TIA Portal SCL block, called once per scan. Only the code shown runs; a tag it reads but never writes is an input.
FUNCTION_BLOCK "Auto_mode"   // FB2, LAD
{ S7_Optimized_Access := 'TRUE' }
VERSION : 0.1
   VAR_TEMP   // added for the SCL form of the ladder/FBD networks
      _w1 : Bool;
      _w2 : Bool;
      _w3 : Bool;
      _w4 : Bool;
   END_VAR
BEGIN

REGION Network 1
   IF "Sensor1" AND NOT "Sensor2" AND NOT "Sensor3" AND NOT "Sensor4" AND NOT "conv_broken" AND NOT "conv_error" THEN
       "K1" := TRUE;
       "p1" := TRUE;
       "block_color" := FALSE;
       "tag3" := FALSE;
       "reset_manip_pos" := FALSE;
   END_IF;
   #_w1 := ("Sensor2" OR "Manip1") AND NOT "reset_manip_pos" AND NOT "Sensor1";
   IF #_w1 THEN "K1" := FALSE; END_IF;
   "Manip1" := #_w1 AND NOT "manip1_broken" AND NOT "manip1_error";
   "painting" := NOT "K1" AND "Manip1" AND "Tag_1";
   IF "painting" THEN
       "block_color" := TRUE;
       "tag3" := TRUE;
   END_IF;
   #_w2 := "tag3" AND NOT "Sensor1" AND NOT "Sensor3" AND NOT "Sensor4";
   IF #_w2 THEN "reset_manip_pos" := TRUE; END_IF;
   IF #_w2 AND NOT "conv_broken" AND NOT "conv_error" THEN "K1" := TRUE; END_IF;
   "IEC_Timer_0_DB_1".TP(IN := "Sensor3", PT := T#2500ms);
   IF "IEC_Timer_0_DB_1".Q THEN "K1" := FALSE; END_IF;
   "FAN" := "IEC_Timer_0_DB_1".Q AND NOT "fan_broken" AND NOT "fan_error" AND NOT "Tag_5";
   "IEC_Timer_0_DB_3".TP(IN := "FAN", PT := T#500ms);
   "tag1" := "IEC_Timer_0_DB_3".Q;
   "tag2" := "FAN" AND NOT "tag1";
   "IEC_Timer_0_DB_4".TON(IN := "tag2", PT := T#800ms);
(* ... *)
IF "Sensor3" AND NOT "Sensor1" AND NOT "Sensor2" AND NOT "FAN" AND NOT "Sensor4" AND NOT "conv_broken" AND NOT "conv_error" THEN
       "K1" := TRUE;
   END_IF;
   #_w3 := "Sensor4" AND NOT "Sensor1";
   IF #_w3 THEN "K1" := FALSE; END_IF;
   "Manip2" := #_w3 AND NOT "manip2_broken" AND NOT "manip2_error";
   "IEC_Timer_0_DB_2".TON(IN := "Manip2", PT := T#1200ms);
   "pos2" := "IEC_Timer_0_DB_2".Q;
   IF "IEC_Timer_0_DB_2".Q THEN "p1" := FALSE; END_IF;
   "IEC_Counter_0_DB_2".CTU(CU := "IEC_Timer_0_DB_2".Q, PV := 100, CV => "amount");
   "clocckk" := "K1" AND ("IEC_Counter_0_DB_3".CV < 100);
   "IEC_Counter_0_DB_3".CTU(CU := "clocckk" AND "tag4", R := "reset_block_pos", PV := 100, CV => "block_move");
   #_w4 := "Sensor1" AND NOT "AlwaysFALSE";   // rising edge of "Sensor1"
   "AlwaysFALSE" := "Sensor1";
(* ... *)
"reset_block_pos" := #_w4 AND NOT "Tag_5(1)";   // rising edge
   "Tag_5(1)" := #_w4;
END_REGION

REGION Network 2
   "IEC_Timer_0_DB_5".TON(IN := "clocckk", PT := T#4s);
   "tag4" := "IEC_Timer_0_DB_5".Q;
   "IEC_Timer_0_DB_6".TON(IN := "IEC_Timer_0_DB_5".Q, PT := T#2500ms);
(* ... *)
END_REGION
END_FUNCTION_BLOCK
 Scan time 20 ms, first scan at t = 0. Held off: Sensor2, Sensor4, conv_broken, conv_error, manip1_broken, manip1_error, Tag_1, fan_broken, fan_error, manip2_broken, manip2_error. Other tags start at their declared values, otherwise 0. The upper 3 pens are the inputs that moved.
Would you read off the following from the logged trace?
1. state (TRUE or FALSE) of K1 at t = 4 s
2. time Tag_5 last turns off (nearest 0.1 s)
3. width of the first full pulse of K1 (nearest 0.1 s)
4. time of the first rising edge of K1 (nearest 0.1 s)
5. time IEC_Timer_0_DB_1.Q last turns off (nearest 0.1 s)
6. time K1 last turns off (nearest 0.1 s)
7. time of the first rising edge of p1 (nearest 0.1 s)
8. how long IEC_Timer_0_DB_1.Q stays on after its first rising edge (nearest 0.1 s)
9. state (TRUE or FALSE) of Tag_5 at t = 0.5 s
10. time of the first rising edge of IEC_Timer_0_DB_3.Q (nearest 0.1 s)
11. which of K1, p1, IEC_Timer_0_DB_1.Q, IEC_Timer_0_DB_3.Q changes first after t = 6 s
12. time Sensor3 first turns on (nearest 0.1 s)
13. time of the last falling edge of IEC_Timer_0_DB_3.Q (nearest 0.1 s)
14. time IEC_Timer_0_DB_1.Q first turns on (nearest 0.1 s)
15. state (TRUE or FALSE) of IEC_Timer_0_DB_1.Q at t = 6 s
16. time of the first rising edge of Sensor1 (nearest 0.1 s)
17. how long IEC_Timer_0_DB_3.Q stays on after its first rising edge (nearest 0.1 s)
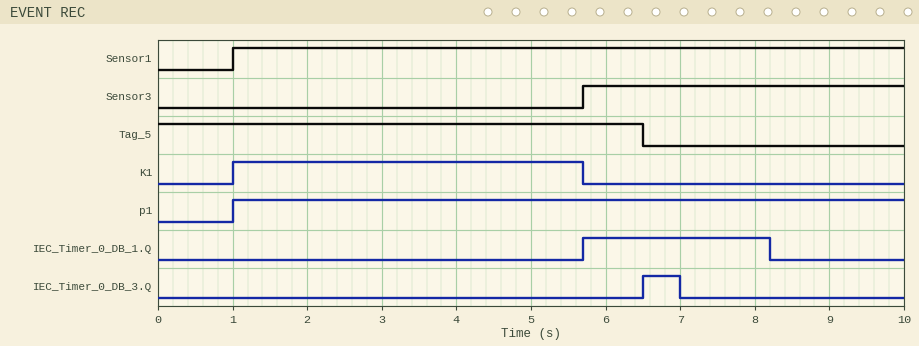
TRUE
6.5 s
4.7 s
1.0 s
8.2 s
5.7 s
1.0 s
2.5 s
TRUE
6.5 s
IEC_Timer_0_DB_3.Q
5.7 s
7.0 s
5.7 s
TRUE
1.0 s
0.5 s
